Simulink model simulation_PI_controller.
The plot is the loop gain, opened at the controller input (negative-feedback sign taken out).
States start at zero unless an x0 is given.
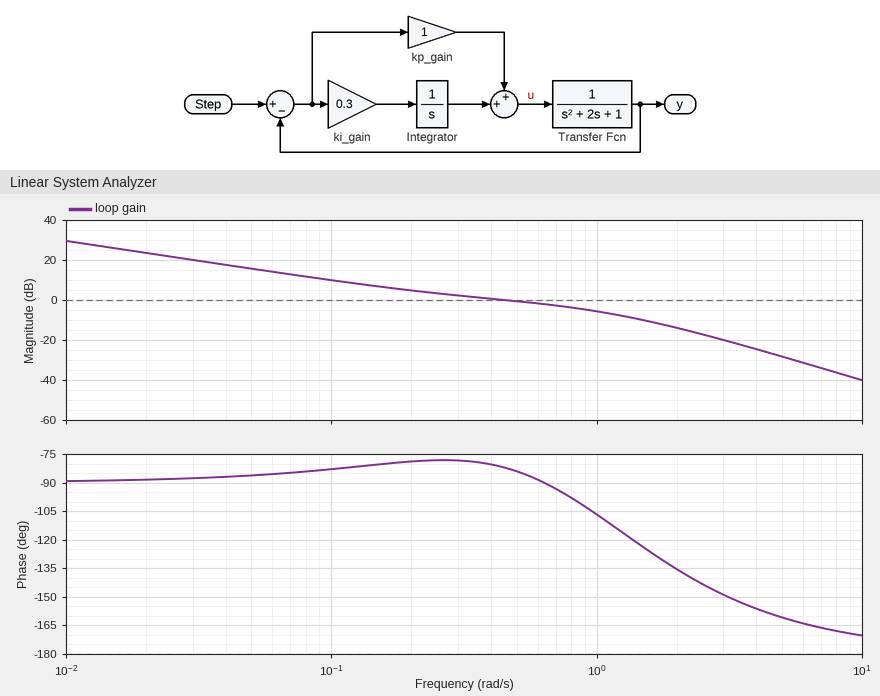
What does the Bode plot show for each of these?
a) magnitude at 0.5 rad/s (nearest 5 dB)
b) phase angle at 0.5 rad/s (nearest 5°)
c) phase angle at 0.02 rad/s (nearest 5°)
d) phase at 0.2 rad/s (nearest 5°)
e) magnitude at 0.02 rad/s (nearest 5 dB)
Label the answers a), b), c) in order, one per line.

a) 0 dB
b) -85°
c) -90°
d) -80°
e) 25 dB
